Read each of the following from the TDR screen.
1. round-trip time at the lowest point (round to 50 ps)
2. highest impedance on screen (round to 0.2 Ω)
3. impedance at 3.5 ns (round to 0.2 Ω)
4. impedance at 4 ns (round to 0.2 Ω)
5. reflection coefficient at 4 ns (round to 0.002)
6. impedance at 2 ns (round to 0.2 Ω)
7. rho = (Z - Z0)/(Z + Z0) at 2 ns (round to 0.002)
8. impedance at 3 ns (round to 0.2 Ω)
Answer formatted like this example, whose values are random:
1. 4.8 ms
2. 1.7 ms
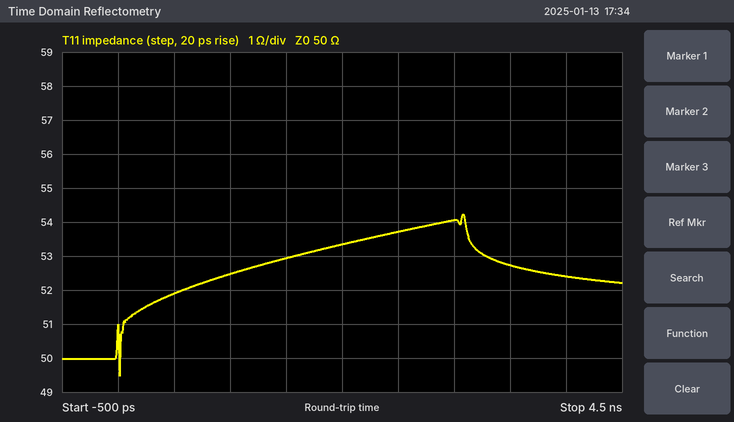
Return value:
1. 0 ps
2. 54.2 Ω
3. 52.8 Ω
4. 52.4 Ω
5. +0.024
6. 53.4 Ω
7. +0.032
8. 54.0 Ω
